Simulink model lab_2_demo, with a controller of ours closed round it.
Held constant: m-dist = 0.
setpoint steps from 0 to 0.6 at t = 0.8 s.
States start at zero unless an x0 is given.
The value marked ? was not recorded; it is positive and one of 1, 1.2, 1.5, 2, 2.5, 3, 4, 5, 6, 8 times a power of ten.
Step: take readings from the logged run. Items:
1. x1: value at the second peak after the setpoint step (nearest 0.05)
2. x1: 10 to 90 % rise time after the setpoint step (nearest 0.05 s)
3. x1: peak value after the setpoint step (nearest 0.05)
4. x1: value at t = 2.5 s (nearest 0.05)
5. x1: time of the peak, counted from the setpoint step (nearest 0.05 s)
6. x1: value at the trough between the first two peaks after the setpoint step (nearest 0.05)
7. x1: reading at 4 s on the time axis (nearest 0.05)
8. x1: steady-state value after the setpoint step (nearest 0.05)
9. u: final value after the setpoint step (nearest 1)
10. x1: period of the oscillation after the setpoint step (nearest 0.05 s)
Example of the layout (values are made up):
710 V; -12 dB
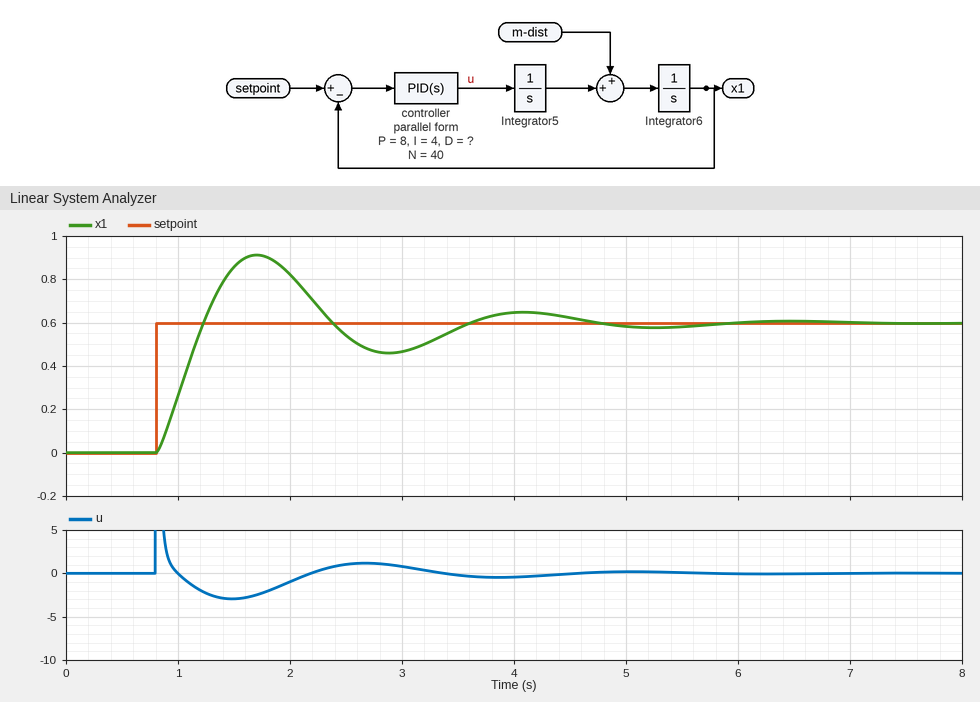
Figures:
0.65; 0.30 s; 0.90; 0.55; 0.90 s; 0.45; 0.65; 0.60; 0; 2.40 s
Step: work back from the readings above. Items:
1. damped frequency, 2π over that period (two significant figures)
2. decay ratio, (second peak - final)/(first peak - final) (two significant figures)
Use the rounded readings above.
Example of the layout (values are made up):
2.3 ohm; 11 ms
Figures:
2.6 rad/s; 0.17
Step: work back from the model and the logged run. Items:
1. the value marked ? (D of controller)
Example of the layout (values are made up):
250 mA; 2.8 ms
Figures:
2
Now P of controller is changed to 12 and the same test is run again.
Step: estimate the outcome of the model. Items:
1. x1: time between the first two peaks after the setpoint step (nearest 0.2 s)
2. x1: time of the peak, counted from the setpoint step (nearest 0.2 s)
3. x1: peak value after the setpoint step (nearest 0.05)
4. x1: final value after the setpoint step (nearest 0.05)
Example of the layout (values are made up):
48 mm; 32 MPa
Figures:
1.8 s; 0.8 s; 0.95; 0.60
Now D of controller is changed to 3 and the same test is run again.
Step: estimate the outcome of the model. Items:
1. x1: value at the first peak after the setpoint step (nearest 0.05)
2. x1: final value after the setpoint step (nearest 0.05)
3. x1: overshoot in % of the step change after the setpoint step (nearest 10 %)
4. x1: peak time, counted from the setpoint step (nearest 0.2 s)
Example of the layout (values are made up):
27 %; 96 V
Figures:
0.80; 0.60; 40 %; 0.8 s
